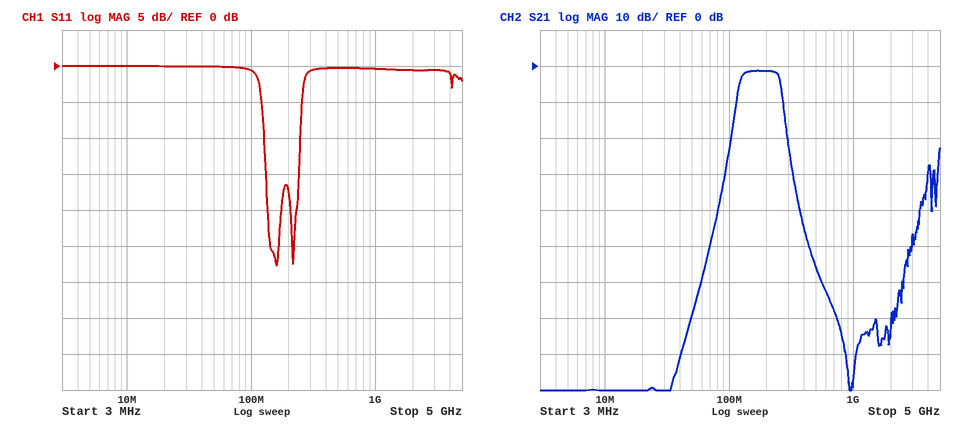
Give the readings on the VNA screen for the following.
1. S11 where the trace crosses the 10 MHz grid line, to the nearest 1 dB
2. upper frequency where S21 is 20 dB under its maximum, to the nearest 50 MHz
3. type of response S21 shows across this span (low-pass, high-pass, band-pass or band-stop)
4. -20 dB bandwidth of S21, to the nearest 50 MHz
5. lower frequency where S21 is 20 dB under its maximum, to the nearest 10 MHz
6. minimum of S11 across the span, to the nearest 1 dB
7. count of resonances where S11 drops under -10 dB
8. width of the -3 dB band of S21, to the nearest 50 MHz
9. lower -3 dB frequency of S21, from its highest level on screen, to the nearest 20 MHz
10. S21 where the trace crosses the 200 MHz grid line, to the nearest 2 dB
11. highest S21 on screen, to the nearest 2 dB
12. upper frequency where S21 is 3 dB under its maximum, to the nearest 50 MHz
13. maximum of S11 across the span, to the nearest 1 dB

0 dB
300 MHz
band-pass
200 MHz
100 MHz
-28 dB
2
150 MHz
120 MHz
-2 dB
-2 dB
250 MHz
0 dB
